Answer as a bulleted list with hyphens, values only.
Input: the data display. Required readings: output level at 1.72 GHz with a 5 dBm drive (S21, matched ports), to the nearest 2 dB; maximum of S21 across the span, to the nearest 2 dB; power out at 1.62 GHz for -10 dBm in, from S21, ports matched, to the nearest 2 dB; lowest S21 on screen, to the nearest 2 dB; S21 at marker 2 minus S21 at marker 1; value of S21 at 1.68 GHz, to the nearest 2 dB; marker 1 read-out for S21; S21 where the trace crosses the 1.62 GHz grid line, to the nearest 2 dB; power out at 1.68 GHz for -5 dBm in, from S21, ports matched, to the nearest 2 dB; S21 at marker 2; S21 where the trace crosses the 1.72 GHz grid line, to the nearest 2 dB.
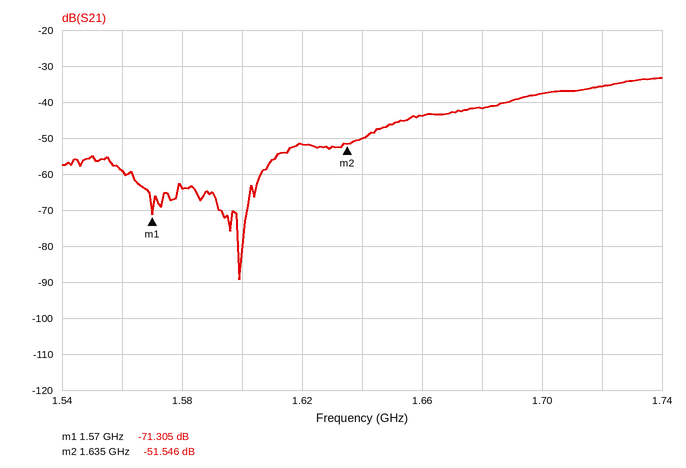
- -30 dBm
- -34 dB
- -62 dBm
- -90 dB
- 19.759 dB
- -42 dB
- -71.305 dB
- -52 dB
- -46 dBm
- -51.546 dB
- -36 dB
